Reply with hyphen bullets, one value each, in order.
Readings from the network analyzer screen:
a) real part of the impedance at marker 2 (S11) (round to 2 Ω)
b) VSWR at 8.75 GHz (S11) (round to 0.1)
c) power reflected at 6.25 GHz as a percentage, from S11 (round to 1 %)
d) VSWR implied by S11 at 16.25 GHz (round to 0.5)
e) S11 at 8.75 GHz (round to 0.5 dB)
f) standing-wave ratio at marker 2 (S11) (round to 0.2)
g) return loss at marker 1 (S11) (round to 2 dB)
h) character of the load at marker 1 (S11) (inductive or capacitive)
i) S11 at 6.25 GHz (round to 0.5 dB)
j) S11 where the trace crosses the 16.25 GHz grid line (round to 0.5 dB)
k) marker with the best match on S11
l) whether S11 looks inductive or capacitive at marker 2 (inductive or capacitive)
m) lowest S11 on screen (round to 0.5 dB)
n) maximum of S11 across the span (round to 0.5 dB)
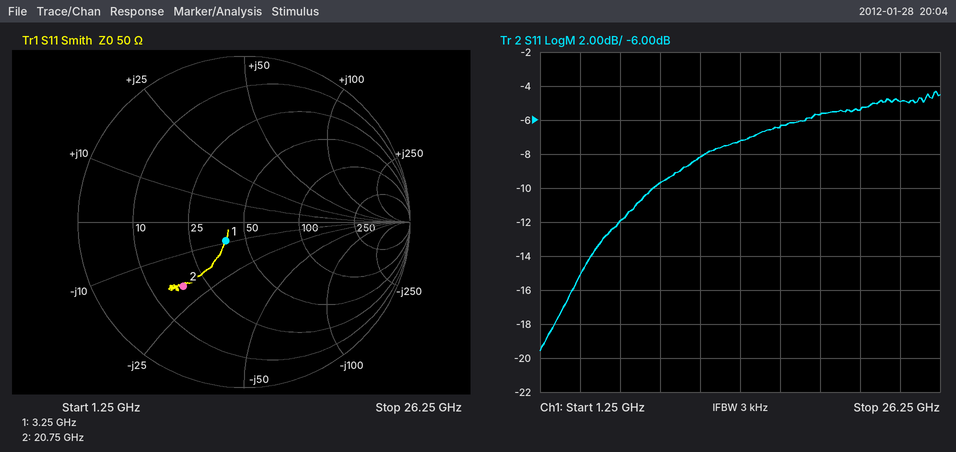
- 18 Ω
- 2.0
- 6 %
- 3.0
- -9.5 dB
- 3.2
- 16 dB
- capacitive
- -12.0 dB
- -6.5 dB
- marker 1
- capacitive
- -19.5 dB
- -4.5 dB
